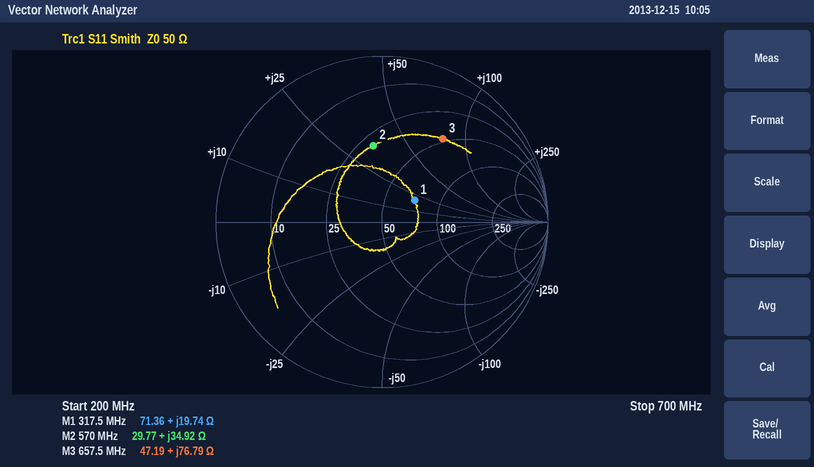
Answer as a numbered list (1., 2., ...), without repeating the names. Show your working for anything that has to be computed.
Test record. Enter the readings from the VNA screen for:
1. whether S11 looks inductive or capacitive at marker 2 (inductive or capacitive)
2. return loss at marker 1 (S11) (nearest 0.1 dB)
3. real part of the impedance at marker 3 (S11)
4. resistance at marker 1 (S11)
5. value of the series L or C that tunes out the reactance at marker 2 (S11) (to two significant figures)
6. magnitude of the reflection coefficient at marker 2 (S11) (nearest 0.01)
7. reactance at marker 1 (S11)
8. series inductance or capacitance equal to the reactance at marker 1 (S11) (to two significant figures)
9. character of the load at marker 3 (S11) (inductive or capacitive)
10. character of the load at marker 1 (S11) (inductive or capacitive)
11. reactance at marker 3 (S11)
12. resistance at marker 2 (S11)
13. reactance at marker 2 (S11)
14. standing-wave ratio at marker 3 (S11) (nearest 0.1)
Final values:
1. inductive
2. 12.5 dB
3. 47.19 Ω
4. 71.36 Ω
5. C = 1/(2π × 570 MHz × 34.92 Ω) ≈ 8.0 pF
6. 0.46
7. +19.74 Ω
8. L = 19.74 Ω/(2π × 317.5 MHz) ≈ 9.9 nH
9. inductive
10. inductive
11. +76.79 Ω
12. 29.77 Ω
13. +34.92 Ω
14. 4.3
